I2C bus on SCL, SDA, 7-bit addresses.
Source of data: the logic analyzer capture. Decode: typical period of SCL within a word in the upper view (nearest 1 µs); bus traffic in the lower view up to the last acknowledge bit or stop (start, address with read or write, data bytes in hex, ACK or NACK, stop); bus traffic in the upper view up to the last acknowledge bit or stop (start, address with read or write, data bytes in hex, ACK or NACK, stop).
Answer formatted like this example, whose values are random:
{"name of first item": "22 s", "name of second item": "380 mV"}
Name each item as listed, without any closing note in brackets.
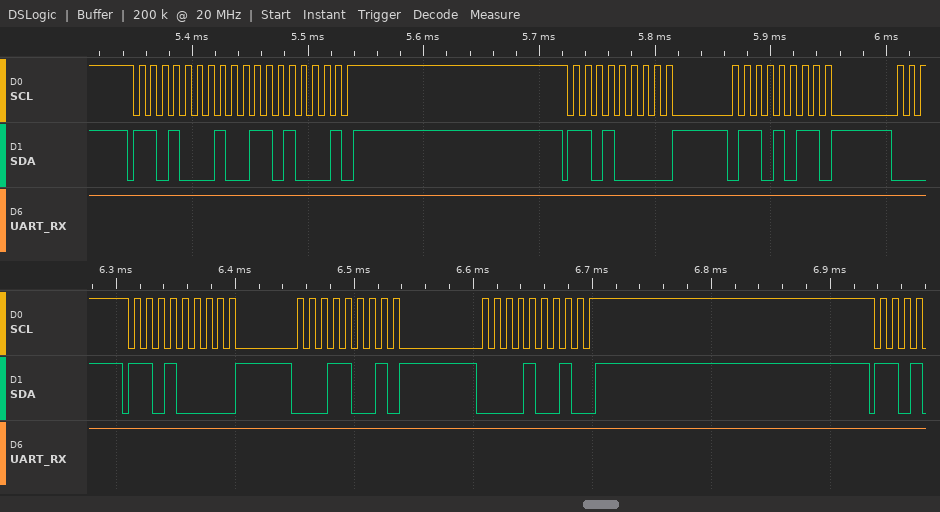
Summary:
{"typical period of SCL within a word in the upper view": "10 µs", "bus traffic in the lower view up to the last acknowledge bit or stop": "start, address 68 write ACK, 19 ACK, 09 ACK, stop", "bus traffic in the upper view up to the last acknowledge bit or stop": "start, address 68 read ACK, 68 NACK, stop, start, address 68 write ACK, 6B ACK"}
